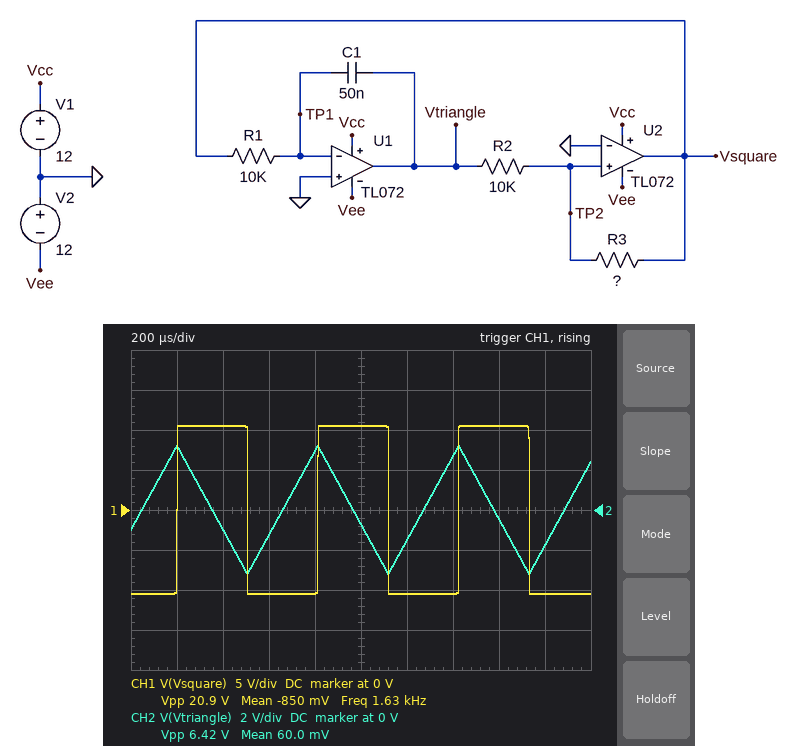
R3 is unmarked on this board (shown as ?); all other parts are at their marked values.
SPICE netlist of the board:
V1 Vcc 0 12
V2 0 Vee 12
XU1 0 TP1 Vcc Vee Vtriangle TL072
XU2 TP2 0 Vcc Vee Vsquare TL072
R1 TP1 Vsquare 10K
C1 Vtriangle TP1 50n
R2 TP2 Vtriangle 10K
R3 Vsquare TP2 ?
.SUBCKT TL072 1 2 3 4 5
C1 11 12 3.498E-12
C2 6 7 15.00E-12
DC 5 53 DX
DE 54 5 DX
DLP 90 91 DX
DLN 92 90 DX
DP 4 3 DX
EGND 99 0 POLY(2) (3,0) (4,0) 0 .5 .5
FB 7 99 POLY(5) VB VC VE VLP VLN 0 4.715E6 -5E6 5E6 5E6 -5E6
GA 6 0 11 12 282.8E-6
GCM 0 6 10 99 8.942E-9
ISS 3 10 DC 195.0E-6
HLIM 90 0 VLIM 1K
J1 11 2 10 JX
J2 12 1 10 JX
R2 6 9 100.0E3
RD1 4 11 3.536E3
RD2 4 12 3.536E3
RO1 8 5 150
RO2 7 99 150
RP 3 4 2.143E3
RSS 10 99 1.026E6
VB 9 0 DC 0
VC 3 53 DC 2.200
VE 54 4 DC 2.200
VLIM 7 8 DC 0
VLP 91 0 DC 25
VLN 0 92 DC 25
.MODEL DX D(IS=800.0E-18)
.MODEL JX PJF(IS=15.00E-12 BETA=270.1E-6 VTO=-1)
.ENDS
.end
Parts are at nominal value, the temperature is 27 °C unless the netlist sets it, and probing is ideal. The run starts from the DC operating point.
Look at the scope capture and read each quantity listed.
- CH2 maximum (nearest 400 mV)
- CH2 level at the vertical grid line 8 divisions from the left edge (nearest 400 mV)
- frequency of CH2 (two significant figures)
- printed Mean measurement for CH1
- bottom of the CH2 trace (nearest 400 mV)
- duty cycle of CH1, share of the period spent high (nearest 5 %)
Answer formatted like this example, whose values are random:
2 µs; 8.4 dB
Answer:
3.2 V; -400 mV; 1.6 kHz; -850 mV; -3.2 V; 50 %
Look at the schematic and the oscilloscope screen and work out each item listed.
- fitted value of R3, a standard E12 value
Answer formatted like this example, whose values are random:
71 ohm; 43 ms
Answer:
33 kΩ
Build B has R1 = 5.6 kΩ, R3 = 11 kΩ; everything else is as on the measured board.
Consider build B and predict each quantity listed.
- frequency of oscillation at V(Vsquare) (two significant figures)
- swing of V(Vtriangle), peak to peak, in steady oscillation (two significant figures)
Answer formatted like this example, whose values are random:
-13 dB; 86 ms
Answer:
980 Hz; 19 V
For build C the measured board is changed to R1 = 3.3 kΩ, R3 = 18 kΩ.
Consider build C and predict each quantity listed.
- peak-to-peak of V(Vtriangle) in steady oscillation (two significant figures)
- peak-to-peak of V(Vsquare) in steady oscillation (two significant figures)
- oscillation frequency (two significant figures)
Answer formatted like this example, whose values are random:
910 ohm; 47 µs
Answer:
12 V; 21 V; 2.7 kHz
